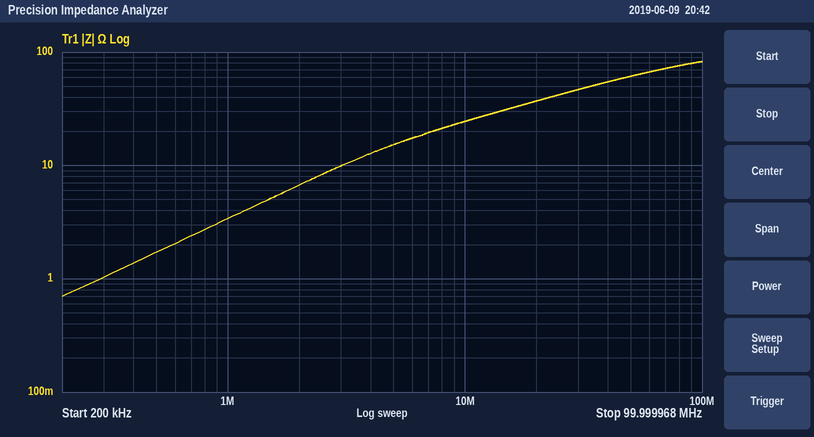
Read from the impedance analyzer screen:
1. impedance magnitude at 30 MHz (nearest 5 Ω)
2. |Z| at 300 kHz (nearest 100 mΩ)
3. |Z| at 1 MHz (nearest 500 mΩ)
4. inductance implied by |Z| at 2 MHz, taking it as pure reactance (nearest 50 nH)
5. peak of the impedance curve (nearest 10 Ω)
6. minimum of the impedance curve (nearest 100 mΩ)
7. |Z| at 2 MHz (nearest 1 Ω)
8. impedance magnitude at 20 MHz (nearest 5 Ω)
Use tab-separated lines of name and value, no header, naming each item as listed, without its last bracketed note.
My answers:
impedance magnitude at 30 MHz	45 Ω
|Z| at 300 kHz	1.0 Ω
|Z| at 1 MHz	3.5 Ω
inductance implied by |Z| at 2 MHz, taking it as pure reactance	550 nH
peak of the impedance curve	80 Ω
minimum of the impedance curve	700 mΩ
|Z| at 2 MHz	7 Ω
impedance magnitude at 20 MHz	35 Ω
